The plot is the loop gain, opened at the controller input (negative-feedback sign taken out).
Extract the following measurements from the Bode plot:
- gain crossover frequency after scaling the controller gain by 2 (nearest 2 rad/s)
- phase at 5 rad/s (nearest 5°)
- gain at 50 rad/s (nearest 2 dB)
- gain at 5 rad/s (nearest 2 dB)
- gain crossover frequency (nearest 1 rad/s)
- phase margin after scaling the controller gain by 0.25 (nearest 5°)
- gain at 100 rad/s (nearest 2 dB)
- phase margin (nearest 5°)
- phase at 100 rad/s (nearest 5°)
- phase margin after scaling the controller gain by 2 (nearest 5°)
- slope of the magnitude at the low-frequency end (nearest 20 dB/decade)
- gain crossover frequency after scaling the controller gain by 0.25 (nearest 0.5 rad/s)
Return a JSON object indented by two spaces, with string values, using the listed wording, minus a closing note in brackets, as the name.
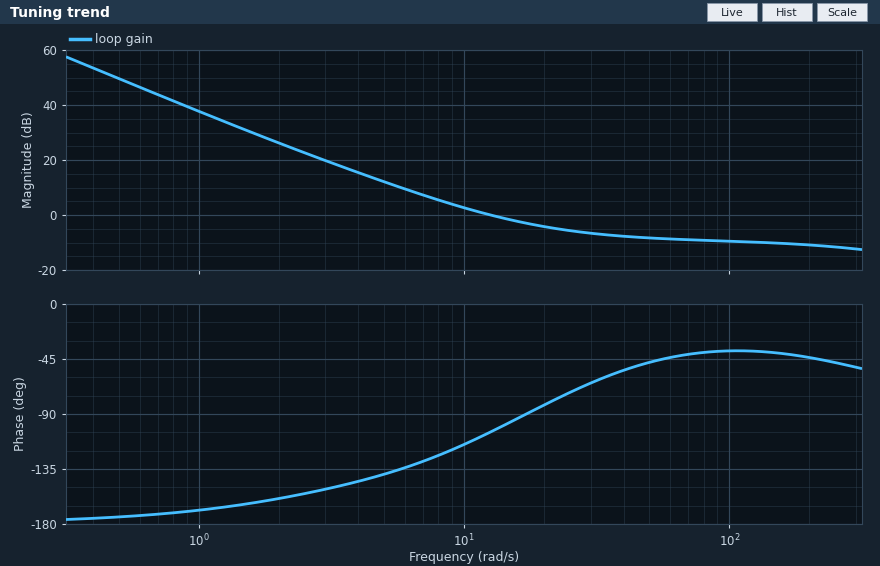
{
  "gain crossover frequency after scaling the controller gain by 2": "26 rad/s",
  "phase at 5 rad/s": "-140°",
  "gain at 50 rad/s": "-8 dB",
  "gain at 5 rad/s": "12 dB",
  "gain crossover frequency": "13 rad/s",
  "phase margin after scaling the controller gain by 0.25": "40°",
  "gain at 100 rad/s": "-10 dB",
  "phase margin": "75°",
  "phase at 100 rad/s": "-40°",
  "phase margin after scaling the controller gain by 2": "110°",
  "slope of the magnitude at the low-frequency end": "-40 dB/decade",
  "gain crossover frequency after scaling the controller gain by 0.25": "5.0 rad/s"
}
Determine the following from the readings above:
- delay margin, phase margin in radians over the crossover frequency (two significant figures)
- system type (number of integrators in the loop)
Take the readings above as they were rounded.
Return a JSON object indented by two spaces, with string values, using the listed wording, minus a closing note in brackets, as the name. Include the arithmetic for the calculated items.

{
  "delay margin, phase margin in radians over the crossover frequency": "75 × π / 180 / 13 = 0.10 s",
  "system type": "2"
}
